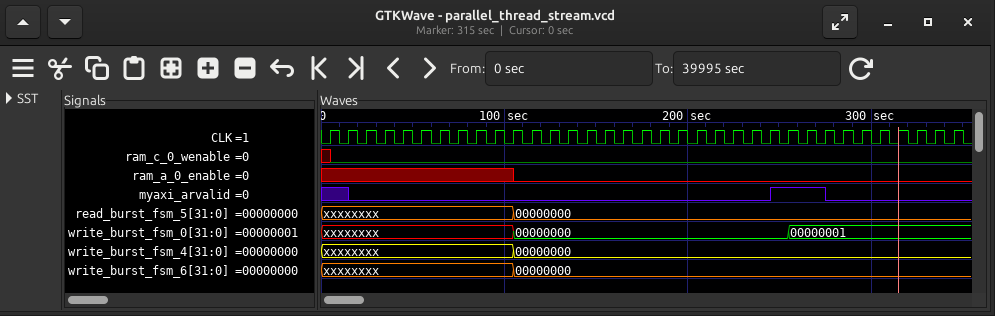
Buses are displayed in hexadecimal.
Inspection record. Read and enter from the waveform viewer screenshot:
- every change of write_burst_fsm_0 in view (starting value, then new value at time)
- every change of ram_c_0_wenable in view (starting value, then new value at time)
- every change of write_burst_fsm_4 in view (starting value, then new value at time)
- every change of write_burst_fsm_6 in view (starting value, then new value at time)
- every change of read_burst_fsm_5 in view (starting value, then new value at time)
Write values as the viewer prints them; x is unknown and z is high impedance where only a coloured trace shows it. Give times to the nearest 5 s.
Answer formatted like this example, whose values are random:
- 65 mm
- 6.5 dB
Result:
- xxxxxxxx, 00000000 at 105 s, 00000001 at 255 s
- x, 0 at 5 s
- xxxxxxxx, 00000000 at 105 s
- xxxxxxxx, 00000000 at 105 s
- xxxxxxxx, 00000000 at 105 s
